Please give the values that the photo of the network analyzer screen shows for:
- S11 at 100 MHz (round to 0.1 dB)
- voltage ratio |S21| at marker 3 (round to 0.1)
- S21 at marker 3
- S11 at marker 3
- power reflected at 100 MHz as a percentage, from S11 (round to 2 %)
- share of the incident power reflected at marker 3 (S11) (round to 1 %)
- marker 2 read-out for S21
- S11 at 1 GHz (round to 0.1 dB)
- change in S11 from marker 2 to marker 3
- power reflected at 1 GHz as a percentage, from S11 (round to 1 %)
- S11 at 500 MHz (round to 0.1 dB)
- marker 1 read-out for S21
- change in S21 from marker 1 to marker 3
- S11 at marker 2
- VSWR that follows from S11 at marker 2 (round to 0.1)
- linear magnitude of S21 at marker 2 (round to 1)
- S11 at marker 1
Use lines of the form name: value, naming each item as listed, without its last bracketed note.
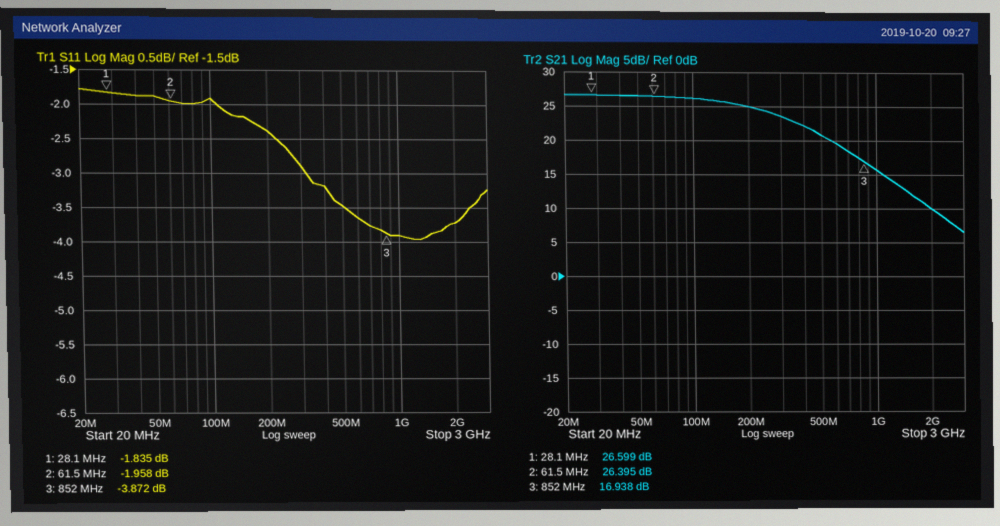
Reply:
S11 at 100 MHz: -1.9 dB
voltage ratio |S21| at marker 3: 7.0
S21 at marker 3: 16.938 dB
S11 at marker 3: -3.872 dB
power reflected at 100 MHz as a percentage, from S11: 64 %
share of the incident power reflected at marker 3 (S11): 41 %
marker 2 read-out for S21: 26.395 dB
S11 at 1 GHz: -3.9 dB
change in S11 from marker 2 to marker 3: -1.914 dB
power reflected at 1 GHz as a percentage, from S11: 41 %
S11 at 500 MHz: -3.5 dB
marker 1 read-out for S21: 26.599 dB
change in S21 from marker 1 to marker 3: -9.661 dB
S11 at marker 2: -1.958 dB
VSWR that follows from S11 at marker 2: 8.9
linear magnitude of S21 at marker 2: 21
S11 at marker 1: -1.835 dB
